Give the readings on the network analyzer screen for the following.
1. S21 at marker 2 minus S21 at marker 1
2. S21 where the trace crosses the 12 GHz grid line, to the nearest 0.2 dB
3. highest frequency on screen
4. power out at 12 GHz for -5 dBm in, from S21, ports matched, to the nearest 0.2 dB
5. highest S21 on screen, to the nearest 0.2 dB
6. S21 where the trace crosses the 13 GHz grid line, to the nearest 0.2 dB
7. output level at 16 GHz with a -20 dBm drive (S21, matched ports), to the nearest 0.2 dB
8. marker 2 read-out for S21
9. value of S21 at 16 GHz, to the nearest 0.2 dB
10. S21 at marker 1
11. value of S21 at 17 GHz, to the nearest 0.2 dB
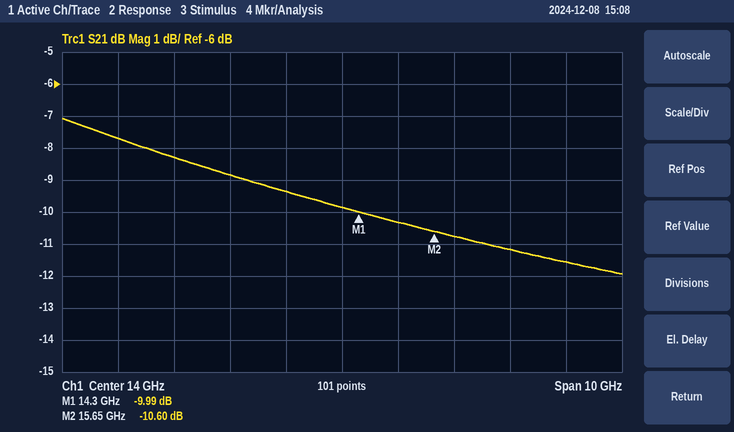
-0.61 dB
-8.8 dB
19 GHz
-13.8 dBm
-7.0 dB
-9.4 dB
-30.8 dBm
-10.60 dB
-10.8 dB
-9.99 dB
-11.2 dB
